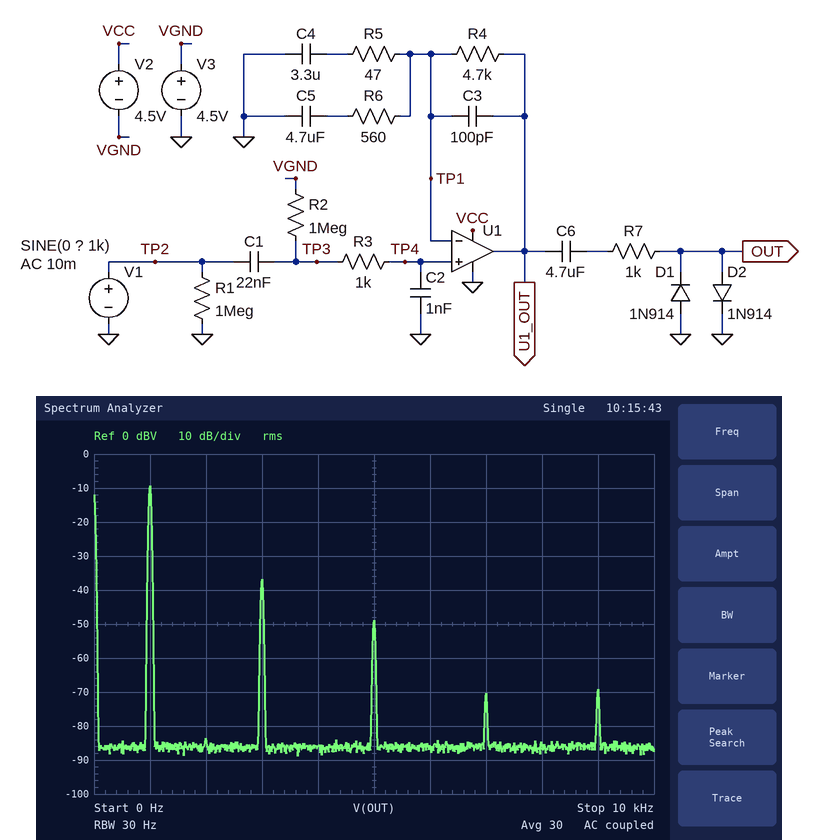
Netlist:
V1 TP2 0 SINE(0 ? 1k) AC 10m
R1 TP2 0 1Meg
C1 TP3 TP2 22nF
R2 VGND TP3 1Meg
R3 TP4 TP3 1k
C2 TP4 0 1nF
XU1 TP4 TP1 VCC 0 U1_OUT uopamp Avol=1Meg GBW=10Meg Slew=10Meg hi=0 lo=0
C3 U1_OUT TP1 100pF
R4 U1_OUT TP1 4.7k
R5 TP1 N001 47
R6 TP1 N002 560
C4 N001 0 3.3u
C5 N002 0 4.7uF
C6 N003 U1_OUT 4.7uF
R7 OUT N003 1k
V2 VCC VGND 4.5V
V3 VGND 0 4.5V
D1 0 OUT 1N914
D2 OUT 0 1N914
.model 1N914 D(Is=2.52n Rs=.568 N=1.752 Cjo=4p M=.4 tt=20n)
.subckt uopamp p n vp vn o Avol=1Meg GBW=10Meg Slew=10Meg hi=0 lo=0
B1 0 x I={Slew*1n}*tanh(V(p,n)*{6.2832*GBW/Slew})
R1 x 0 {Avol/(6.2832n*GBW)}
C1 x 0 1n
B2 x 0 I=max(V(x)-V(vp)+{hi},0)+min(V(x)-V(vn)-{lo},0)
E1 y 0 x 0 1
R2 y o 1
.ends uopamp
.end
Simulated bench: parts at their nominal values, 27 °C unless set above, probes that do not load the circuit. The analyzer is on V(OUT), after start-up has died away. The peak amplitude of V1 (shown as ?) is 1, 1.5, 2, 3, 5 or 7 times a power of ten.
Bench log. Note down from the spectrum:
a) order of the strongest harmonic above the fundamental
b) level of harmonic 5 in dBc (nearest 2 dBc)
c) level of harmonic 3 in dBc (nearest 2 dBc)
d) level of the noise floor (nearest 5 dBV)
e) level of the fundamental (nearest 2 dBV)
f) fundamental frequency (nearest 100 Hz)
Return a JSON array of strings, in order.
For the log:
["3", "-40 dBc", "-28 dBc", "-85 dBV", "-10 dBV", "1.0 kHz"]
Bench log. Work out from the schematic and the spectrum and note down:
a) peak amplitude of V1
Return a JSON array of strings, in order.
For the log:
["7 mV"]
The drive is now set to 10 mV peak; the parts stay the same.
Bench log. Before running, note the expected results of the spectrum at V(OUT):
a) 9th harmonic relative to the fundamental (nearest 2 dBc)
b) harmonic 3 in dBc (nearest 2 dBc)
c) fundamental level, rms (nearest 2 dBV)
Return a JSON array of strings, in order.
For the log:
["-50 dBc", "-18 dBc", "-8 dBV"]
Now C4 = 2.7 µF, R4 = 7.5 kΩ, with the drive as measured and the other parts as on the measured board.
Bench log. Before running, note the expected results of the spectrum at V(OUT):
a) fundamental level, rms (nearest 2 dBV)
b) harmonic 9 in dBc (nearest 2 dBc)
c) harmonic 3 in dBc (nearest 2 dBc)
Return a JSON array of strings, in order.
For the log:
["-8 dBV", "-50 dBc", "-18 dBc"]
